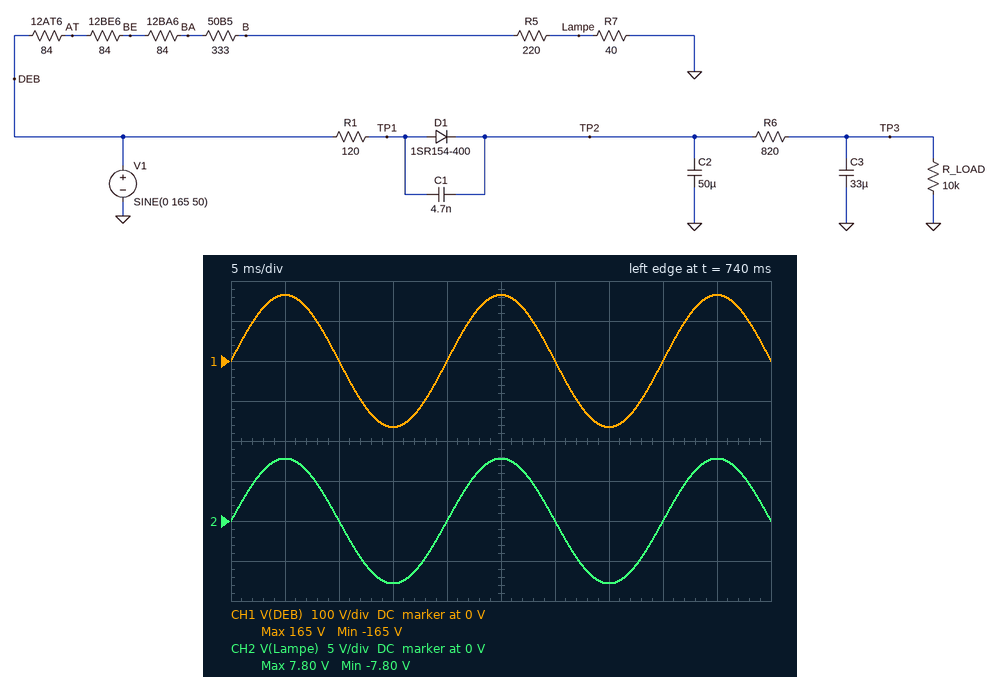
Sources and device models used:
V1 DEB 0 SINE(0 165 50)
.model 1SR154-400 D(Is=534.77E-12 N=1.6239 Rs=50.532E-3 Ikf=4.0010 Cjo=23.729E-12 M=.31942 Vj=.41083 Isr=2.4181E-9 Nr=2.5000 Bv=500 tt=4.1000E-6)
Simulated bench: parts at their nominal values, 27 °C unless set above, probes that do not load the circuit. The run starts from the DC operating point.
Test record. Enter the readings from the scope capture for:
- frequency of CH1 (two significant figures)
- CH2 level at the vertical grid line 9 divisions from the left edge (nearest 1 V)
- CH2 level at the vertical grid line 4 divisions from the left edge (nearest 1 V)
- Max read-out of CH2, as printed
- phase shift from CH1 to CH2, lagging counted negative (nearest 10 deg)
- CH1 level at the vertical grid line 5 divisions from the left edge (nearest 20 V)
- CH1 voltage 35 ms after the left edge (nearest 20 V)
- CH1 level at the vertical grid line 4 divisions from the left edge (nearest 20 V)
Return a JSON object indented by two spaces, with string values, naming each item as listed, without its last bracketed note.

{
  "frequency of CH1": "50 Hz",
  "CH2 level at the vertical grid line 9 divisions from the left edge": "8 V",
  "CH2 level at the vertical grid line 4 divisions from the left edge": "0 V",
  "Max read-out of CH2, as printed": "7.80 V",
  "phase shift from CH1 to CH2, lagging counted negative": "0 deg",
  "CH1 level at the vertical grid line 5 divisions from the left edge": "160 V",
  "CH1 voltage 35 ms after the left edge": "-160 V",
  "CH1 level at the vertical grid line 4 divisions from the left edge": "0 V"
}
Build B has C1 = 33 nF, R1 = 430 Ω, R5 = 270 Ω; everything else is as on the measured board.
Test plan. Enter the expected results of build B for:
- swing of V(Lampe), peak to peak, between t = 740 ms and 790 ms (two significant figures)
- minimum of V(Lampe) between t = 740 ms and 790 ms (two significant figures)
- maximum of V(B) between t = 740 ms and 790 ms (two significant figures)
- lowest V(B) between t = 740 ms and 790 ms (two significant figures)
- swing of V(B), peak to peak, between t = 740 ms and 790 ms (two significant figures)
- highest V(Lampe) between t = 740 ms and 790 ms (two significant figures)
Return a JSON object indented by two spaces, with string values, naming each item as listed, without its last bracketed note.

{
  "swing of V(Lampe), peak to peak, between t = 740 ms and 790 ms": "15 V",
  "minimum of V(Lampe) between t = 740 ms and 790 ms": "-7.4 V",
  "maximum of V(B) between t = 740 ms and 790 ms": "57 V",
  "lowest V(B) between t = 740 ms and 790 ms": "-57 V",
  "swing of V(B), peak to peak, between t = 740 ms and 790 ms": "110 V",
  "highest V(Lampe) between t = 740 ms and 790 ms": "7.4 V"
}
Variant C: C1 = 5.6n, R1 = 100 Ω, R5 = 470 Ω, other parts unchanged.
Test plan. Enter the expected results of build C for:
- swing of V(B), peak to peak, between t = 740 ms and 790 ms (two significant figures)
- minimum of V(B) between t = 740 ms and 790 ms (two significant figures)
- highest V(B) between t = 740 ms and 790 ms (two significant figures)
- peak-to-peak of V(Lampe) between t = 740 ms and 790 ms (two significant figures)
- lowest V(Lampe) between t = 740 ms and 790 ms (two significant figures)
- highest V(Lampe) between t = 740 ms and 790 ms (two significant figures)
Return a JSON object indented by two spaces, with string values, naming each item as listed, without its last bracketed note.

{
  "swing of V(B), peak to peak, between t = 740 ms and 790 ms": "150 V",
  "minimum of V(B) between t = 740 ms and 790 ms": "-77 V",
  "highest V(B) between t = 740 ms and 790 ms": "77 V",
  "peak-to-peak of V(Lampe) between t = 740 ms and 790 ms": "12 V",
  "lowest V(Lampe) between t = 740 ms and 790 ms": "-6.0 V",
  "highest V(Lampe) between t = 740 ms and 790 ms": "6.0 V"
}
